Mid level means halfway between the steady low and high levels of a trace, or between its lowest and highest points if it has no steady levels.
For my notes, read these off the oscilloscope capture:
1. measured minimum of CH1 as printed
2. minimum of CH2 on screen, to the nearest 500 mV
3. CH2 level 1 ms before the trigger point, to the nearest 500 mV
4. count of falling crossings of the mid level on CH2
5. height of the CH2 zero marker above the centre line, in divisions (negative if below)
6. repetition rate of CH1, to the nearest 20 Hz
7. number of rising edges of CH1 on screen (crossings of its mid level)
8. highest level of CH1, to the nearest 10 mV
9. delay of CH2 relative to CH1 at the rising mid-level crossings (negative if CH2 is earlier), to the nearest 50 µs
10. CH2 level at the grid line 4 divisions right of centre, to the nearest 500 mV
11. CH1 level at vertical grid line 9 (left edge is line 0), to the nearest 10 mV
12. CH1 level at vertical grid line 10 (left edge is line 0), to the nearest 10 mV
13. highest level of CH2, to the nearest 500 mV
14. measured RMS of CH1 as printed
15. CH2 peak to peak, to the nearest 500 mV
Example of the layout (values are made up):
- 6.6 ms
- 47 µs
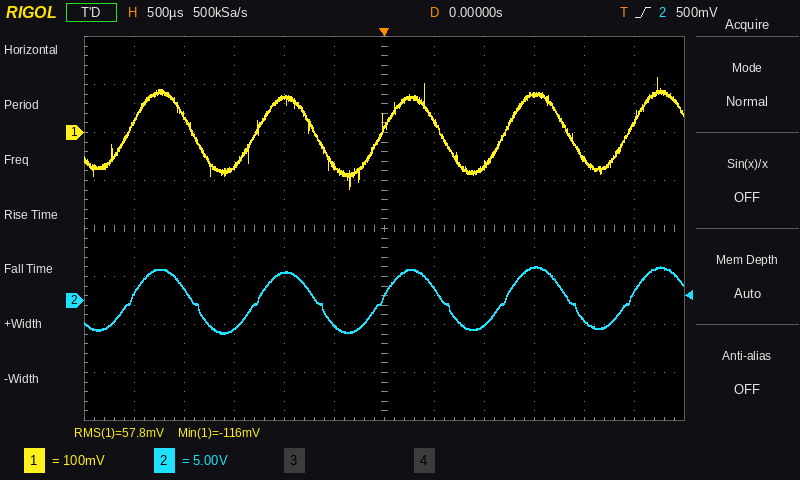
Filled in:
- -116 mV
- -3.5 V
- 3.0 V
- 4
- -1.5 div
- 800 Hz
- 5
- 110 mV
- 0 µs
- -2.0 V
- 80 mV
- -60 mV
- 3.5 V
- 57.8 mV
- 7.0 V
